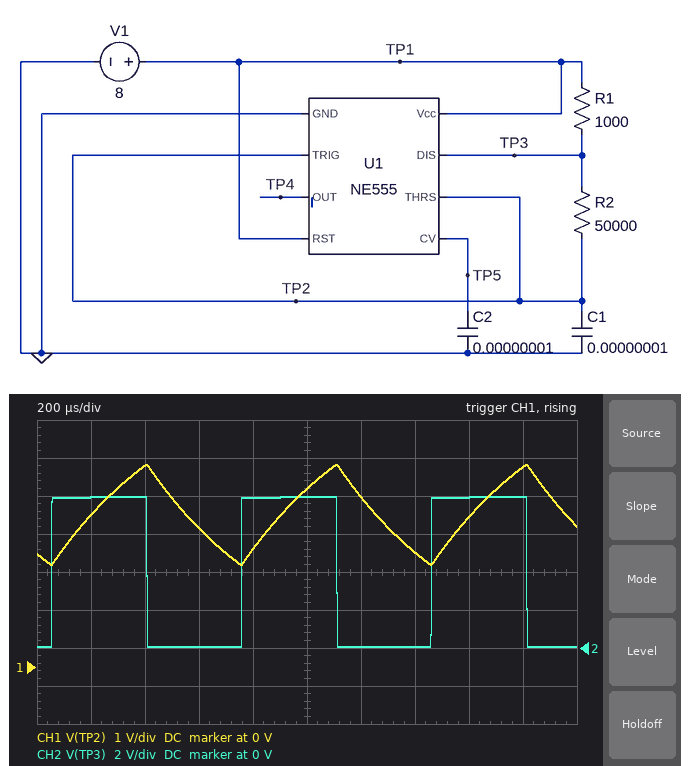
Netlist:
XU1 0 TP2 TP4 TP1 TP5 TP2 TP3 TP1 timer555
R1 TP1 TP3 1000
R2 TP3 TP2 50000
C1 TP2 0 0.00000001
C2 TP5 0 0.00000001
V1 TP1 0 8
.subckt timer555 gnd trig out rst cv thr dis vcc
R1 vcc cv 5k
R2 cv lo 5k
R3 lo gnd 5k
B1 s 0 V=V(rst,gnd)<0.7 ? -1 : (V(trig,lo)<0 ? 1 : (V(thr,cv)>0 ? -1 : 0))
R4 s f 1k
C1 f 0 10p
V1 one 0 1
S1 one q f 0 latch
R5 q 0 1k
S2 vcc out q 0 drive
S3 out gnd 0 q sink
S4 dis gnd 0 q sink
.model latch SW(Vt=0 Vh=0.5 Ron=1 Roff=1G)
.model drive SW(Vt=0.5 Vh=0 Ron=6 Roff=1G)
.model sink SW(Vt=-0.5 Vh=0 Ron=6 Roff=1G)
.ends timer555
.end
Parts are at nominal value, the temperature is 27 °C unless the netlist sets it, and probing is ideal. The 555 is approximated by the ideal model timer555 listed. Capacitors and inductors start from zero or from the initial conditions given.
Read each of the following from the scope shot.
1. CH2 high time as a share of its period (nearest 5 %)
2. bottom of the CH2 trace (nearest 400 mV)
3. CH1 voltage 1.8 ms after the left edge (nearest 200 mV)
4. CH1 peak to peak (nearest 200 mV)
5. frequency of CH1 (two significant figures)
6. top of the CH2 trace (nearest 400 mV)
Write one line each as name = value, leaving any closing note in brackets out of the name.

CH2 high time as a share of its period = 50 %
bottom of the CH2 trace = 0 V
CH1 voltage 1.8 ms after the left edge = 5.2 V
CH1 peak to peak = 2.6 V
frequency of CH1 = 1.4 kHz
top of the CH2 trace = 8.0 V
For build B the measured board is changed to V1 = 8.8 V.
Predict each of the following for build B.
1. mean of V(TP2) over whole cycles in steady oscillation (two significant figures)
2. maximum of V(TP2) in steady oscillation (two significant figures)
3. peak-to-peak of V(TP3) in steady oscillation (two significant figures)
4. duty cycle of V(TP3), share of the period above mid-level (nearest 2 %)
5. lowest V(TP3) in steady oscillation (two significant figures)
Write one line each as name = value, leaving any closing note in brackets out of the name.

mean of V(TP2) over whole cycles in steady oscillation = 4.4 V
maximum of V(TP2) in steady oscillation = 5.9 V
peak-to-peak of V(TP3) in steady oscillation = 8.7 V
duty cycle of V(TP3), share of the period above mid-level = 50 %
lowest V(TP3) in steady oscillation = 53 mV
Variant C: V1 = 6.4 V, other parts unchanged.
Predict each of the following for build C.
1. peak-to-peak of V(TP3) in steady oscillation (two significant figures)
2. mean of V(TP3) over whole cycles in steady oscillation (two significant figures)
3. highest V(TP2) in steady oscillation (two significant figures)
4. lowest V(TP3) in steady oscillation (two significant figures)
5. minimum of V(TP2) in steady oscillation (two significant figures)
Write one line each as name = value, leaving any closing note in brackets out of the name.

peak-to-peak of V(TP3) in steady oscillation = 6.3 V
mean of V(TP3) over whole cycles in steady oscillation = 3.2 V
highest V(TP2) in steady oscillation = 4.3 V
lowest V(TP3) in steady oscillation = 38 mV
minimum of V(TP2) in steady oscillation = 2.1 V
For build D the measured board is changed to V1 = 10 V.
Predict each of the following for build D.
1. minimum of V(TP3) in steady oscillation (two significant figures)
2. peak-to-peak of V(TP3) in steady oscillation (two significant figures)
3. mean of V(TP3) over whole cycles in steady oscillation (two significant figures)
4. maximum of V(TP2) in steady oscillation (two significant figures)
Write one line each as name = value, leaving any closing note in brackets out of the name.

minimum of V(TP3) in steady oscillation = 60 mV
peak-to-peak of V(TP3) in steady oscillation = 9.9 V
mean of V(TP3) over whole cycles in steady oscillation = 5.0 V
maximum of V(TP2) in steady oscillation = 6.7 V
